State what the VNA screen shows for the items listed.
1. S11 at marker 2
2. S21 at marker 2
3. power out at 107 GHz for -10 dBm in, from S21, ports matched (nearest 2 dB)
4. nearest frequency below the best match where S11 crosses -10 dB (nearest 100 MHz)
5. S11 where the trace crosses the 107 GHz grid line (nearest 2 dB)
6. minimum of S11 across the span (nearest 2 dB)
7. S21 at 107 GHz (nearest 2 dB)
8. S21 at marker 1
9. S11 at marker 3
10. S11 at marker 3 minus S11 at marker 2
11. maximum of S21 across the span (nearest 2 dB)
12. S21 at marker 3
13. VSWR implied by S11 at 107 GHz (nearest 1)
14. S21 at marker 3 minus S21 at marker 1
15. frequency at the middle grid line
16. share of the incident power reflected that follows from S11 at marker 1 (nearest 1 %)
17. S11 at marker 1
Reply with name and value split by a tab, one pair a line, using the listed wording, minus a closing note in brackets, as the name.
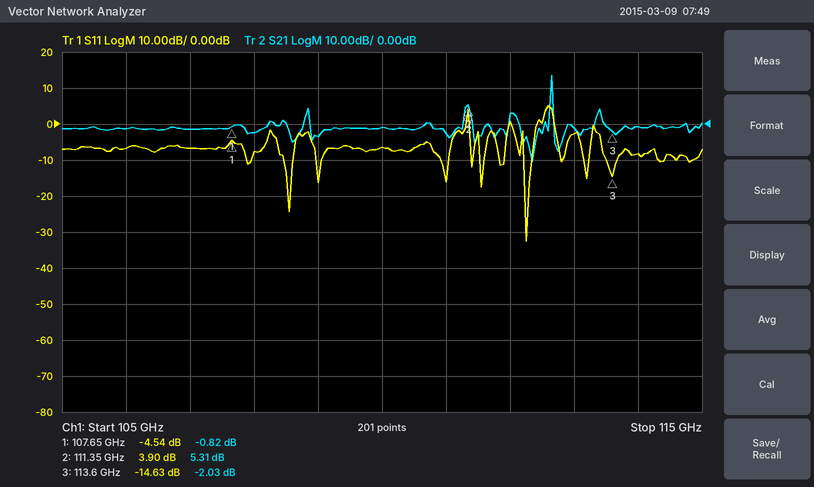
S11 at marker 2	3.90 dB
S21 at marker 2	5.31 dB
power out at 107 GHz for -10 dBm in, from S21, ports matched	-12 dBm
nearest frequency below the best match where S11 crosses -10 dB	112.2 GHz
S11 where the trace crosses the 107 GHz grid line	-6 dB
minimum of S11 across the span	-32 dB
S21 at 107 GHz	-2 dB
S21 at marker 1	-0.82 dB
S11 at marker 3	-14.63 dB
S11 at marker 3 minus S11 at marker 2	-18.53 dB
maximum of S21 across the span	14 dB
S21 at marker 3	-2.03 dB
VSWR implied by S11 at 107 GHz	3
S21 at marker 3 minus S21 at marker 1	-1.21 dB
frequency at the middle grid line	110 GHz
share of the incident power reflected that follows from S11 at marker 1	35 %
S11 at marker 1	-4.54 dB
